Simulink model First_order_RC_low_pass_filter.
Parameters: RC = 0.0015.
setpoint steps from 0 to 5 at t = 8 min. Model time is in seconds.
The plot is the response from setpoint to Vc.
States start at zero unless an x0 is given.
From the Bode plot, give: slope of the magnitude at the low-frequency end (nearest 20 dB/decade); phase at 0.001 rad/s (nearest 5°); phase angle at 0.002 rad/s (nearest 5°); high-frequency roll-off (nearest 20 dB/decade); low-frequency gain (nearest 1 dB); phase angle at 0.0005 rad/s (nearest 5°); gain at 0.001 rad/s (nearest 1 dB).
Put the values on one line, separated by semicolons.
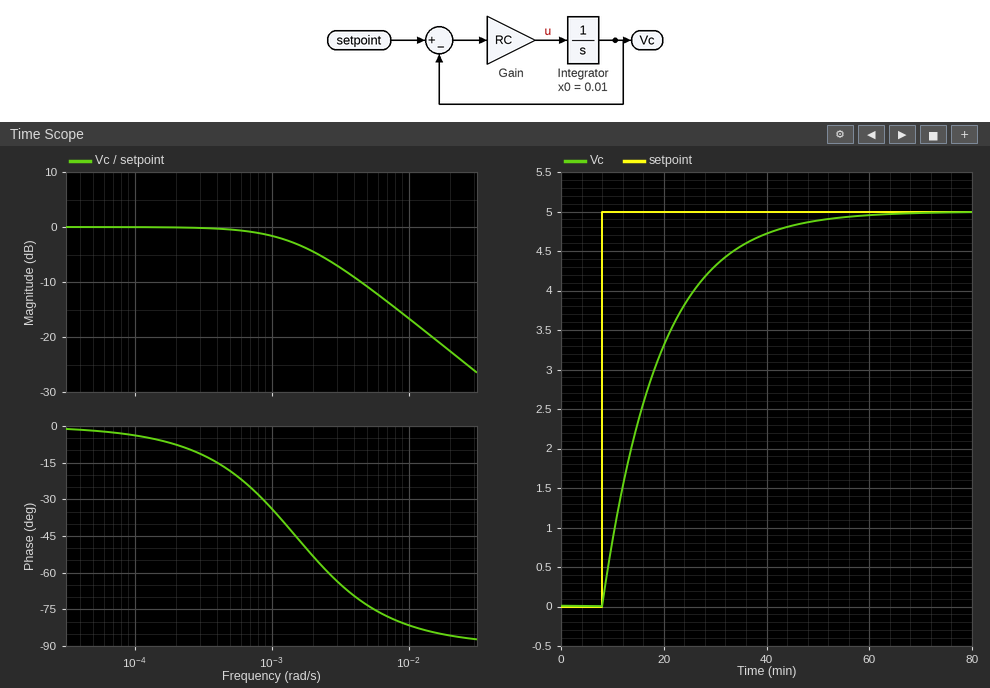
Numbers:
0 dB/decade; -35°; -55°; -20 dB/decade; 0 dB; -20°; -2 dB
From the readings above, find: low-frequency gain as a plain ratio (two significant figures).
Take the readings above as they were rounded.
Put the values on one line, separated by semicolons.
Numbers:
1.0
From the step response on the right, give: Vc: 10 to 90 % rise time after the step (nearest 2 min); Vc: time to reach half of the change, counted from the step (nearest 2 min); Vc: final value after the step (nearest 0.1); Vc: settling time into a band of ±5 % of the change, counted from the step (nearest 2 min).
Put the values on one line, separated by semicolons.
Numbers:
24 min; 8 min; 5.0; 34 min
